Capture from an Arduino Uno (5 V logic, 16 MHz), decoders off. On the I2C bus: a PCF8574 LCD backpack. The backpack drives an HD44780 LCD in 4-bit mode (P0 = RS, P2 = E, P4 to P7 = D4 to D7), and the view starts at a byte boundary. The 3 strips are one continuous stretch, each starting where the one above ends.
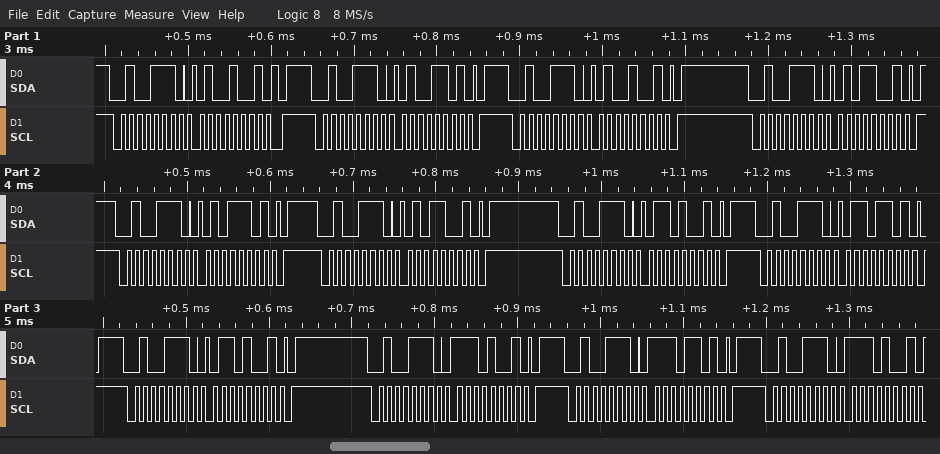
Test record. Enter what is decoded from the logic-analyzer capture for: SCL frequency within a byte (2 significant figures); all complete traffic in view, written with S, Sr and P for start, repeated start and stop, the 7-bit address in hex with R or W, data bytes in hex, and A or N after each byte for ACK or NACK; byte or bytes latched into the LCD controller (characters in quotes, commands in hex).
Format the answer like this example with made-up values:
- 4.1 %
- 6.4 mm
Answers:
- 100 kHz
- S 27W A 49 A P S 27W A 4D A P S 27W A 49 A P S 27W A 59 A P S 27W A 5D A P S 27W A 59 A P S 27W A 69 A P S 27W A 6D A P S 27W A 69 A P S 27W A E9 A P S 27W A ED A P S 27W A E9 A
- 'E' 'n'
